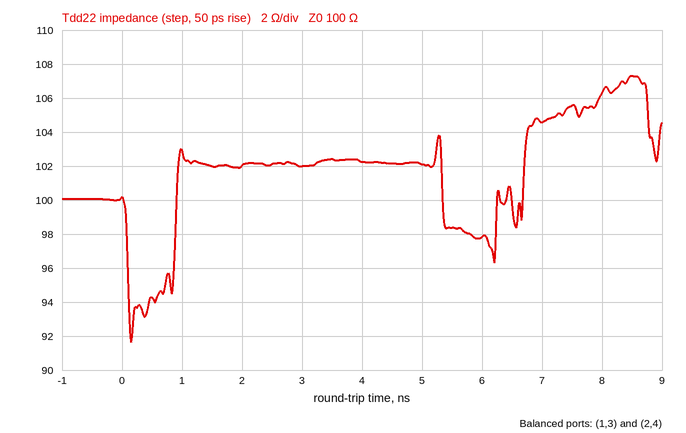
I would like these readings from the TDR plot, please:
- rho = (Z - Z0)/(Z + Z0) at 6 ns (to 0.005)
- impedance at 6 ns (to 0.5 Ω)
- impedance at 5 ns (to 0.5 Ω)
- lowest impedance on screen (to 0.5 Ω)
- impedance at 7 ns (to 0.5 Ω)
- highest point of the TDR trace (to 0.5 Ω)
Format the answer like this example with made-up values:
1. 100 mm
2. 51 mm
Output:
1. -0.010
2. 98.0 Ω
3. 102.0 Ω
4. 91.5 Ω
5. 104.5 Ω
6. 107.5 Ω
